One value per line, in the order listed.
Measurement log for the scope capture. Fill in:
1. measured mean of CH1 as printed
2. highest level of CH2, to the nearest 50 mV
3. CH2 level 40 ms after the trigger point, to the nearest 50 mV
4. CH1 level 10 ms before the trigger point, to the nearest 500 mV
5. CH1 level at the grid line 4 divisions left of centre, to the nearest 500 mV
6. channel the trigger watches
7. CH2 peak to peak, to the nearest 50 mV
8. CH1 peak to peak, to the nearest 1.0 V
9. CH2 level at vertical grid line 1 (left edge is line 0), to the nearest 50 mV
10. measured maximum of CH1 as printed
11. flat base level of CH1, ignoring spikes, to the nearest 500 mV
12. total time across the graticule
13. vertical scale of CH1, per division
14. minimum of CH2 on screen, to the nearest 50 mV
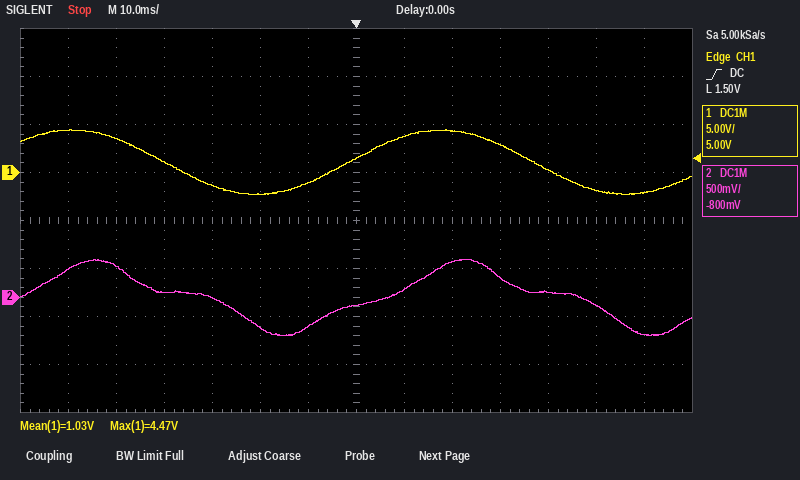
1.03 V
400 mV
50 mV
-1.0 V
1.0 V
CH1
800 mV
7.0 V
300 mV
4.47 V
-2.0 V
140 ms
5 V
-400 mV
